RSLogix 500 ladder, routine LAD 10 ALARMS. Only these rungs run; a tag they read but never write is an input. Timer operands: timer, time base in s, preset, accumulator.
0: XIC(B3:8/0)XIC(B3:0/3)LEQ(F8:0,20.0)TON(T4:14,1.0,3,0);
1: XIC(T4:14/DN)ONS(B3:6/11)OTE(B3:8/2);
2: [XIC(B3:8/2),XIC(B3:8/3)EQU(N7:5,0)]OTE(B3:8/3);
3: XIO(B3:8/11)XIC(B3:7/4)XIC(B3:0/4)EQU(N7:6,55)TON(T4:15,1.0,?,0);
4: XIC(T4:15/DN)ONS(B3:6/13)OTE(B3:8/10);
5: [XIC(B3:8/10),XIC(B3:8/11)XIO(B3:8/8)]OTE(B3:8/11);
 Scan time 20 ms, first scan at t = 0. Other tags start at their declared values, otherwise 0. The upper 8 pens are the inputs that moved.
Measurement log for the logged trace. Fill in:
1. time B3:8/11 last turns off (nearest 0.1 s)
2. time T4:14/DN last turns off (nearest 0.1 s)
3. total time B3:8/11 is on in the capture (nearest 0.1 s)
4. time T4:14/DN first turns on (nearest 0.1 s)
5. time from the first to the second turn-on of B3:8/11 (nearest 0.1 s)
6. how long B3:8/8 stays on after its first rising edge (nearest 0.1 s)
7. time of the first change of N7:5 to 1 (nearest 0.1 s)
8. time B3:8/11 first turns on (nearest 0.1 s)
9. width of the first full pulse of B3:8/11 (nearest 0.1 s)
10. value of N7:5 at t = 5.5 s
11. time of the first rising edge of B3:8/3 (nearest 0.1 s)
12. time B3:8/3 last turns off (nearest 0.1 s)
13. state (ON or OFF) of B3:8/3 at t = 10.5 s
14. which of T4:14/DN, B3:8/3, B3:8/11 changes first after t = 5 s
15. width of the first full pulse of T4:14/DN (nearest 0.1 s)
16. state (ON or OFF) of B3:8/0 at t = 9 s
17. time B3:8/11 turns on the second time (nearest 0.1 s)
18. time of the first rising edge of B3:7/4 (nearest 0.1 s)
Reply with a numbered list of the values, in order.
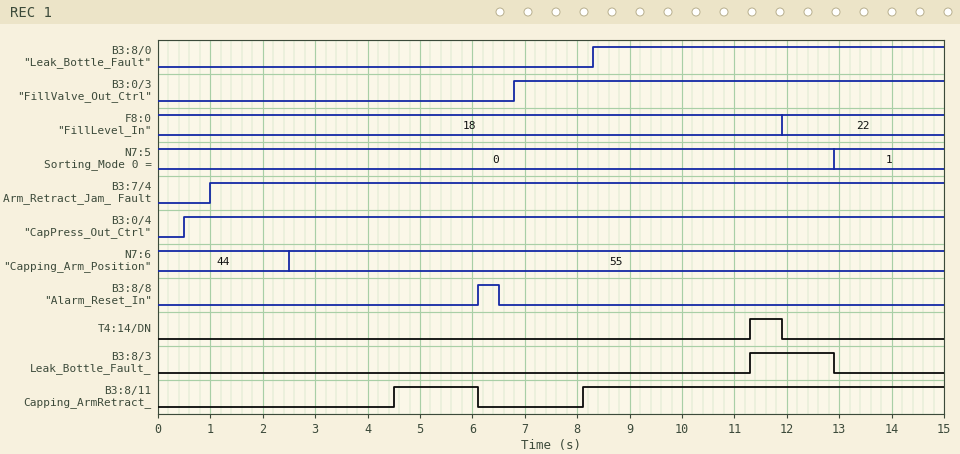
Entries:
1. 6.1 s
2. 11.9 s
3. 8.5 s
4. 11.3 s
5. 3.6 s
6. 0.4 s
7. 12.9 s
8. 4.5 s
9. 1.6 s
10. 0
11. 11.3 s
12. 12.9 s
13. OFF
14. B3:8/11
15. 0.6 s
16. ON
17. 8.1 s
18. 1.0 s
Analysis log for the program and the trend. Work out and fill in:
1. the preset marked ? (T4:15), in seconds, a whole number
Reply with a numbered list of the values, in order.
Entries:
1. 2 s
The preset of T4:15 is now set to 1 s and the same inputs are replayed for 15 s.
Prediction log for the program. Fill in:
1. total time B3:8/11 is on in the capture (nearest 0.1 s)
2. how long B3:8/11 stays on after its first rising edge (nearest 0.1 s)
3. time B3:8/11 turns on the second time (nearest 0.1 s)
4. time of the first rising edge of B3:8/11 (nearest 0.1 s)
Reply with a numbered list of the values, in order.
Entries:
1. 10.5 s
2. 2.6 s
3. 7.1 s
4. 3.5 s
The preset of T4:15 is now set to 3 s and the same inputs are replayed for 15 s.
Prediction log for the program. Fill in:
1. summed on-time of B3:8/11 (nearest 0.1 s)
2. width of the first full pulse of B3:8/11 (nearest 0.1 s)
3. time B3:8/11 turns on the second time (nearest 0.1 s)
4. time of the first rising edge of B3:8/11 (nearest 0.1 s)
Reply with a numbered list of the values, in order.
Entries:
1. 6.5 s
2. 0.6 s
3. 9.1 s
4. 5.5 s
